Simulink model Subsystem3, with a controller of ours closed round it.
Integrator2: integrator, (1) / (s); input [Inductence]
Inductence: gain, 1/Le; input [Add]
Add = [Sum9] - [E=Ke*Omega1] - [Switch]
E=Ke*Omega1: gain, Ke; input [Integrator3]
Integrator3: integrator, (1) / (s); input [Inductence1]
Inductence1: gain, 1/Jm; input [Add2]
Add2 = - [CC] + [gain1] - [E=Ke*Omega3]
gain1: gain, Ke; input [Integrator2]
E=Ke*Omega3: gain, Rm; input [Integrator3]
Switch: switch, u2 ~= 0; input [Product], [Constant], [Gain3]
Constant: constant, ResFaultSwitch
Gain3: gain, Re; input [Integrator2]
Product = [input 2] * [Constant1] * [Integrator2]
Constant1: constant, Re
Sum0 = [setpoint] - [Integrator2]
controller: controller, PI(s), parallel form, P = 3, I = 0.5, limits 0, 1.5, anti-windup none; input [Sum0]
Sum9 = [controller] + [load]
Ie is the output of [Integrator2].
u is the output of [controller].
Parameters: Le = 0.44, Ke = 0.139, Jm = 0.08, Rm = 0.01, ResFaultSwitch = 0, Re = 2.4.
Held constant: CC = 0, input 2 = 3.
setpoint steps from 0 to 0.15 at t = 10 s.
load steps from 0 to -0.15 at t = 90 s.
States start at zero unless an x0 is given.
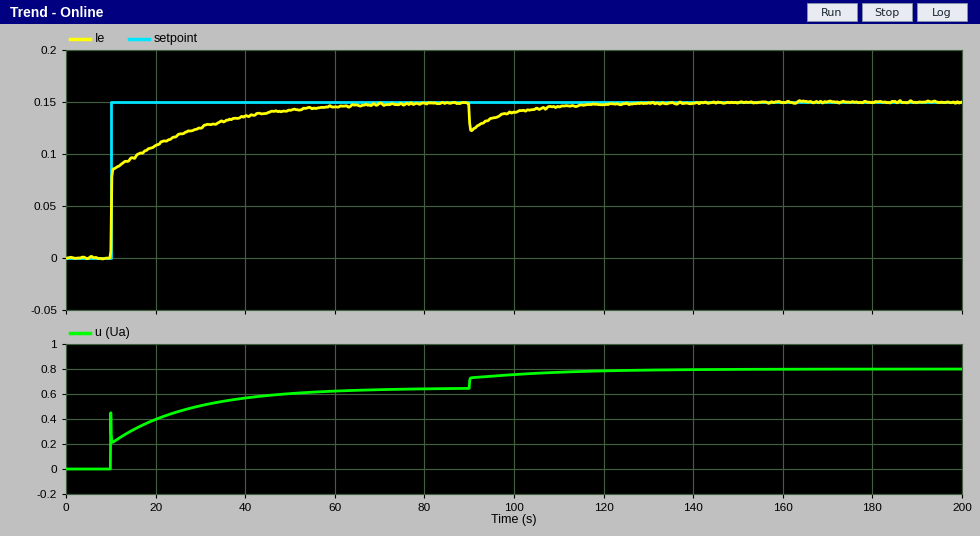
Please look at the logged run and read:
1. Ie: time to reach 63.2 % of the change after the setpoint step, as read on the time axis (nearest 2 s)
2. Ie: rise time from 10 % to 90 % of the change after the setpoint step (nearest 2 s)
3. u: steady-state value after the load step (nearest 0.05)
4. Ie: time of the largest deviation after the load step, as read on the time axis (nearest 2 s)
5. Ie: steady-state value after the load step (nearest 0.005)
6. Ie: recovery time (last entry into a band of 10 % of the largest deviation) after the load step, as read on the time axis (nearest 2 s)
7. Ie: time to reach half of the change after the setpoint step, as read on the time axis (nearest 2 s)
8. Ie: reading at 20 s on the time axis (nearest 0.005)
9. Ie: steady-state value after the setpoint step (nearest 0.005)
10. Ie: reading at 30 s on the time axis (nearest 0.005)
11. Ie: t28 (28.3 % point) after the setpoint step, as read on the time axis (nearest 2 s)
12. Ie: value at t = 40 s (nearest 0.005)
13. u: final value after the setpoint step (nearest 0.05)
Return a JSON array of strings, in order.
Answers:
["14 s", "28 s", "0.80", "90 s", "0.150", "120 s", "10 s", "0.110", "0.150", "0.125", "10 s", "0.135", "0.65"]
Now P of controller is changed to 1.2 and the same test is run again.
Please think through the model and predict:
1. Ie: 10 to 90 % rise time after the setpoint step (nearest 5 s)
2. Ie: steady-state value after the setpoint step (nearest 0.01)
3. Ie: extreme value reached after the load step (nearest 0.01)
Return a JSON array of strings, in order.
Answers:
["25 s", "0.15", "0.11"]
